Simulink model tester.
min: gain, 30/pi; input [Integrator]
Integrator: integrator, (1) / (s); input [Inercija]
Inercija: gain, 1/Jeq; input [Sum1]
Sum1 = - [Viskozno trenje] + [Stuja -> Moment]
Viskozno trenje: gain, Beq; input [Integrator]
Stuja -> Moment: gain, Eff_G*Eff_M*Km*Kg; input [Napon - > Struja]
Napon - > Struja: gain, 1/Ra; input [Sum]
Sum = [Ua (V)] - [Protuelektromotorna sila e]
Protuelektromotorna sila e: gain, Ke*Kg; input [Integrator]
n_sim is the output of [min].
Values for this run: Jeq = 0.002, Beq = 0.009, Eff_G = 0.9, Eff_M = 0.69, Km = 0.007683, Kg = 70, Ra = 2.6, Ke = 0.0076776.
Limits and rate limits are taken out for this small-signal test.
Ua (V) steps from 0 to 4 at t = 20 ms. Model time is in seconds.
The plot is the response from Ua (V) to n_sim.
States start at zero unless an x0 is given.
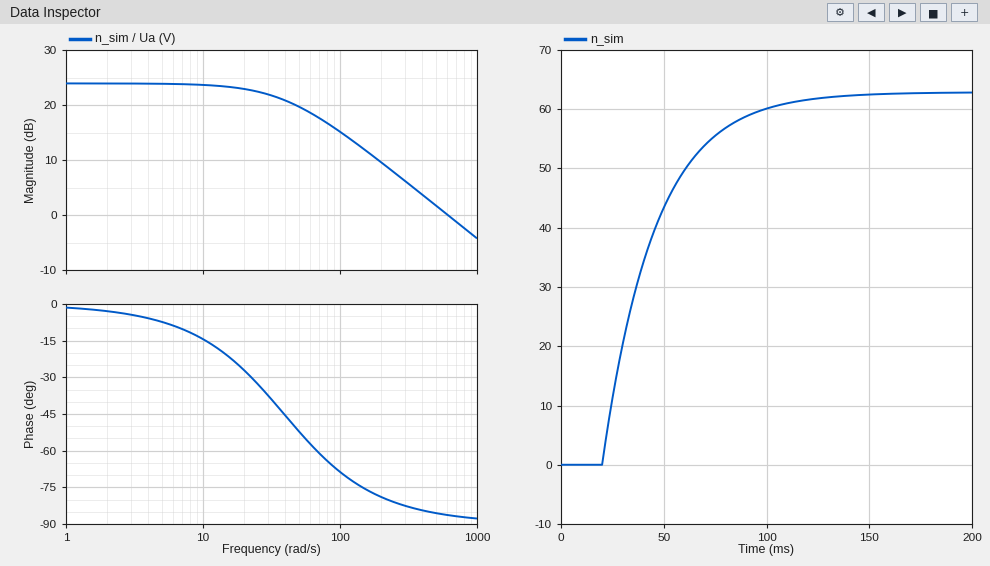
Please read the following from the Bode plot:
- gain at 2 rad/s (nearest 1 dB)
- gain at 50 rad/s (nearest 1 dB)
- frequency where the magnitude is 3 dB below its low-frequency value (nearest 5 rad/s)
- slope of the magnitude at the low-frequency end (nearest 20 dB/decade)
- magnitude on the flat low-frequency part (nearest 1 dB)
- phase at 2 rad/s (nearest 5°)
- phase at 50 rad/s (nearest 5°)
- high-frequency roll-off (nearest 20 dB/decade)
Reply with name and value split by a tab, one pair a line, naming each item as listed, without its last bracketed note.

gain at 2 rad/s	24 dB
gain at 50 rad/s	20 dB
frequency where the magnitude is 3 dB below its low-frequency value	40 rad/s
slope of the magnitude at the low-frequency end	0 dB/decade
magnitude on the flat low-frequency part	24 dB
phase at 2 rad/s	-5°
phase at 50 rad/s	-50°
high-frequency roll-off	-20 dB/decade
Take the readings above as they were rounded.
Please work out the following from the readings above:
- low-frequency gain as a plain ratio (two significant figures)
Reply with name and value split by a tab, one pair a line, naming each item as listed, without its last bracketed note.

low-frequency gain as a plain ratio	16
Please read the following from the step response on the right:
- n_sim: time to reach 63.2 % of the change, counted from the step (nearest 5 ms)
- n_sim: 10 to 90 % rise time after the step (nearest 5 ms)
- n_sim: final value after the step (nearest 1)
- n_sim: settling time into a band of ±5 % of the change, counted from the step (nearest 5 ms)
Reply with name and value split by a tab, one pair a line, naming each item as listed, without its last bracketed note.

n_sim: time to reach 63.2 % of the change, counted from the step	25 ms
n_sim: 10 to 90 % rise time after the step	55 ms
n_sim: final value after the step	63
n_sim: settling time into a band of ±5 % of the change, counted from the step	75 ms
